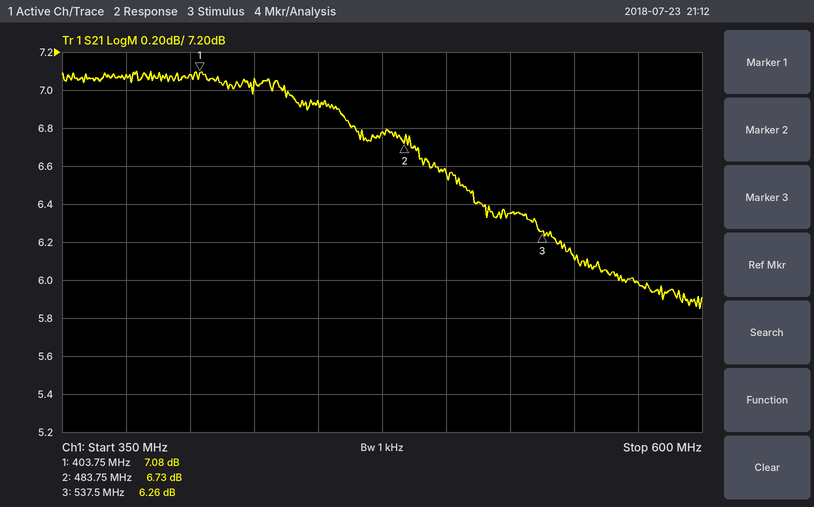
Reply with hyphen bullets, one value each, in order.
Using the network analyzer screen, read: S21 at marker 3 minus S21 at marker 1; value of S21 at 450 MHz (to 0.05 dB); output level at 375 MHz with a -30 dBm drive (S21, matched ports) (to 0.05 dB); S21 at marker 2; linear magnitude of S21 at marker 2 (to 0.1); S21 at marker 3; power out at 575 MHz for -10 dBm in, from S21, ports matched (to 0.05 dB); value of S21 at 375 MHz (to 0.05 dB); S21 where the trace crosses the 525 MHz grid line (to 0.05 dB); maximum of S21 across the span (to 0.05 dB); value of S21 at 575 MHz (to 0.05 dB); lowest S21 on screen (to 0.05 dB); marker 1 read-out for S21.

- -0.82 dB
- 6.95 dB
- -22.90 dBm
- 6.73 dB
- 2.2
- 6.26 dB
- -4.00 dBm
- 7.10 dB
- 6.35 dB
- 7.10 dB
- 6.00 dB
- 5.85 dB
- 7.08 dB
